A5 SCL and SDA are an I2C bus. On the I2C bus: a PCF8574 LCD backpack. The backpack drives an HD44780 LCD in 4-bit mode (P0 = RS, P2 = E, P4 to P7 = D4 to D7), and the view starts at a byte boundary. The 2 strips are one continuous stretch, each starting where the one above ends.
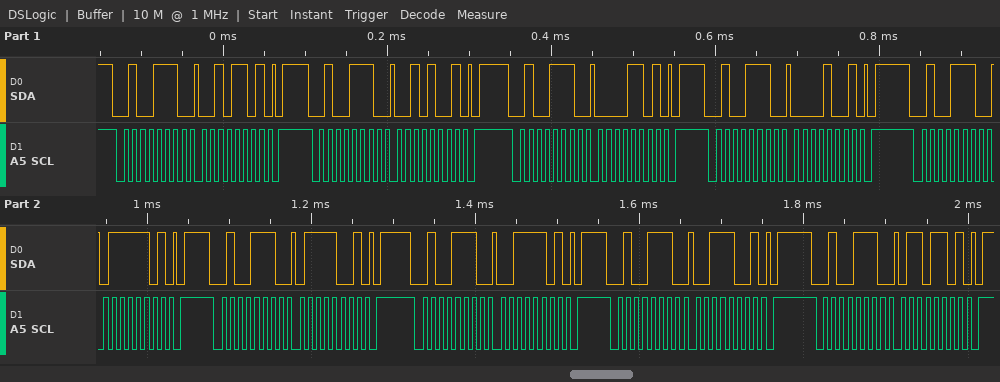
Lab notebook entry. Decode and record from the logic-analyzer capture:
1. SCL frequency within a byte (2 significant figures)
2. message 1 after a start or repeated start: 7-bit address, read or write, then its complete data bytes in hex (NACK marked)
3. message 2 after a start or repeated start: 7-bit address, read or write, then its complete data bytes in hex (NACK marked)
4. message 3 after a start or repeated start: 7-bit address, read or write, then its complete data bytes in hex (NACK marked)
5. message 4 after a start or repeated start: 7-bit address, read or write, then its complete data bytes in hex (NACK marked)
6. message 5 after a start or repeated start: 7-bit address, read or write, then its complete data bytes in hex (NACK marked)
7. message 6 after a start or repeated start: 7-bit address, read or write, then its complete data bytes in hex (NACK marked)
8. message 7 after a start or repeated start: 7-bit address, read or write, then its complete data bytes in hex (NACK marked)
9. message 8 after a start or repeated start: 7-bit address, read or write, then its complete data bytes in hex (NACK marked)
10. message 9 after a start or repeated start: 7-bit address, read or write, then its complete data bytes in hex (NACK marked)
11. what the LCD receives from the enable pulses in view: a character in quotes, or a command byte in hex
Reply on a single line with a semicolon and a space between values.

100 kHz; 0x27 write: 2D; 0x27 write: 29; 0x27 write: 0D; 0x27 write: 09; 0x27 write: 7D; 0x27 write: 79; 0x27 write: 3D; 0x27 write: 39; 0x27 write: 6D; ' ' 's'
